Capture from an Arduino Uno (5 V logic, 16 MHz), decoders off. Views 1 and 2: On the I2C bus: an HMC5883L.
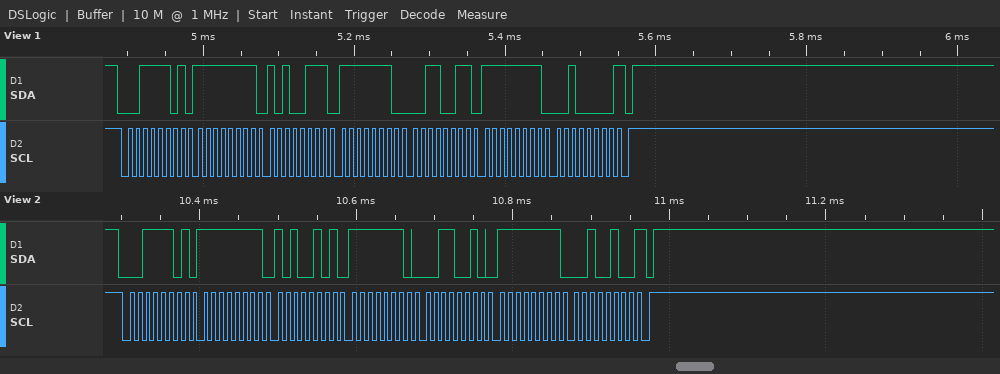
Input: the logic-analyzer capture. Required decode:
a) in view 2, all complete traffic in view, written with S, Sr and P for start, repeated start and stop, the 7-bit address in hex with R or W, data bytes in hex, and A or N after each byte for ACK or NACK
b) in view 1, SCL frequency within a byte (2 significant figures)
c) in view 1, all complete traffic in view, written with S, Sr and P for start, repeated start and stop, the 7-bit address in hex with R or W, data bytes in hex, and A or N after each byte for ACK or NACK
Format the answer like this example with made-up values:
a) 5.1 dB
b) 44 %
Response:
a) S 1ER A FF A A5 A FE A 32 A FF A 24 N P
b) 100 kHz
c) S 1ER A FF A A7 A FE A 33 A FF A 20 N P
